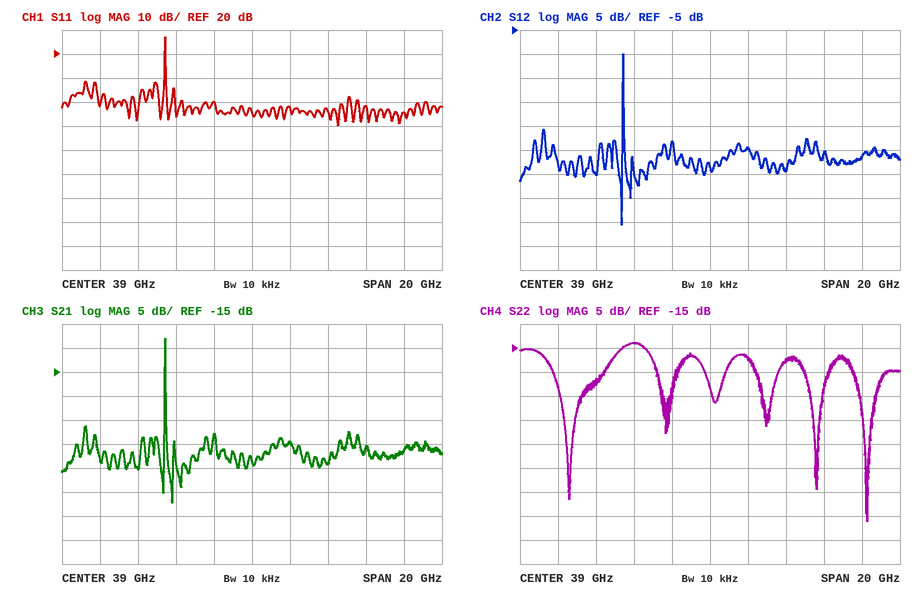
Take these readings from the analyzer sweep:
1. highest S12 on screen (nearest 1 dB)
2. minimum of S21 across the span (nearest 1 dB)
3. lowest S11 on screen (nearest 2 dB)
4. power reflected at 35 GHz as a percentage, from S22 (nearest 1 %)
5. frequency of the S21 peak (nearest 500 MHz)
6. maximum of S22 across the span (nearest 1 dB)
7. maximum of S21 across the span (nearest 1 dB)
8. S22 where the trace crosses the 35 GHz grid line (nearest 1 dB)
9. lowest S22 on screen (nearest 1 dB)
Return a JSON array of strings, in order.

["-10 dB", "-42 dB", "-10 dB", "4 %", "34.5 GHz", "-14 dB", "-8 dB", "-14 dB", "-51 dB"]
